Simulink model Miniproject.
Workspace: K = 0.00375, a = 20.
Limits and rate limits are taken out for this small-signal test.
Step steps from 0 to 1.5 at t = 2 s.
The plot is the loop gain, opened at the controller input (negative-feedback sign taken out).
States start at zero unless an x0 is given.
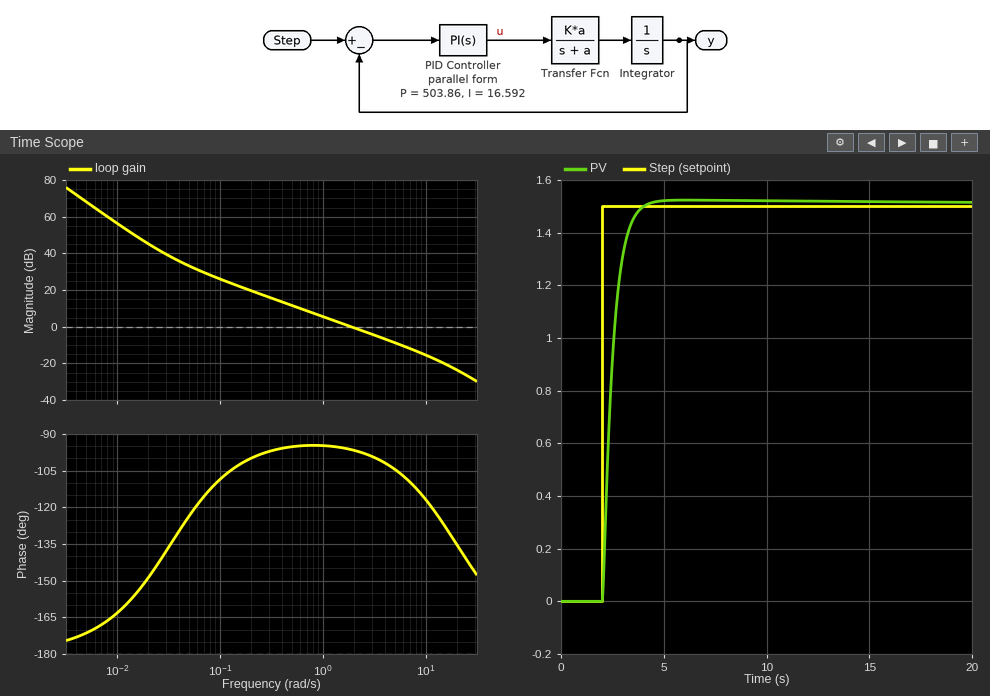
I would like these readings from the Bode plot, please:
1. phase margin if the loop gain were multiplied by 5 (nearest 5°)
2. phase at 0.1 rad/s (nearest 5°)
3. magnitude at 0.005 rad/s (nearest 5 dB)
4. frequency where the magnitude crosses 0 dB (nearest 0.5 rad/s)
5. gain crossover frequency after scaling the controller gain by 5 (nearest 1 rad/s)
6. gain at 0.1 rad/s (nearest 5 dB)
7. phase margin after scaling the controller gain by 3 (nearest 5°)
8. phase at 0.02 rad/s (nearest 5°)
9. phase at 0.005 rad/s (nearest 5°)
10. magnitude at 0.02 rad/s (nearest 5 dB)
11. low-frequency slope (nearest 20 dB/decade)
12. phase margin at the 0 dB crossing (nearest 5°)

65°
-110°
70 dB
2.0 rad/s
9 rad/s
25 dB
75°
-150°
-170°
45 dB
-40 dB/decade
85°
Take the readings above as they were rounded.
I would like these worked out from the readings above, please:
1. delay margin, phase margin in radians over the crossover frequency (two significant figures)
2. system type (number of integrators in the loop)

0.74 s
2
